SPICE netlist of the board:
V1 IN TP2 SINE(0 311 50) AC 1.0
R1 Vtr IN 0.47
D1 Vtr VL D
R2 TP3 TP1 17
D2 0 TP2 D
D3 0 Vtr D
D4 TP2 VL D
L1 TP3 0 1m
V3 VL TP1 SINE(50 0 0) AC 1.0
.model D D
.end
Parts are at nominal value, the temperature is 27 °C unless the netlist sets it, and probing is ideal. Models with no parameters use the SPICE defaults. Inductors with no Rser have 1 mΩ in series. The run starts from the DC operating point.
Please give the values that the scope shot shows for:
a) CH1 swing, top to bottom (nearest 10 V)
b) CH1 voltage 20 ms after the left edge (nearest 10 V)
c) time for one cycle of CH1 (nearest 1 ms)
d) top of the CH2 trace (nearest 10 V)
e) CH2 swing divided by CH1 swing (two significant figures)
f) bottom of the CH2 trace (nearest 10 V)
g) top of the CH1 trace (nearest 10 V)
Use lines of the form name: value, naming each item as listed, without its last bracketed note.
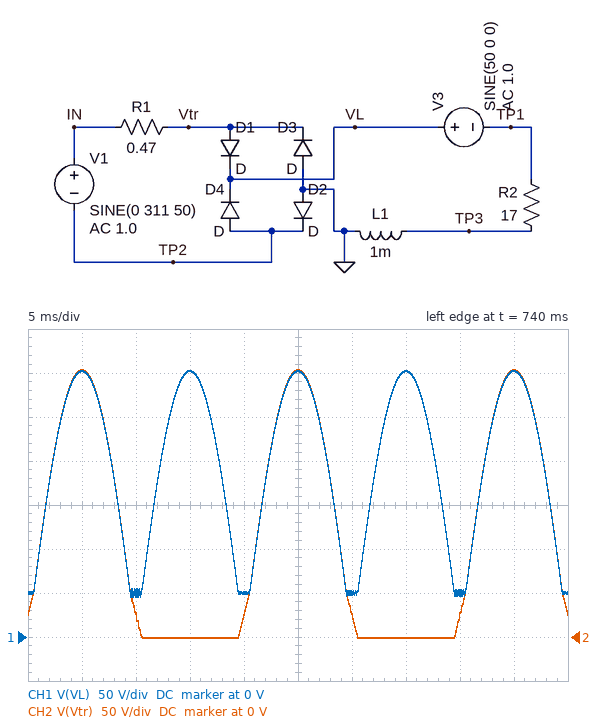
CH1 swing, top to bottom: 260 V
CH1 voltage 20 ms after the left edge: 50 V
time for one cycle of CH1: 10 ms
top of the CH2 trace: 300 V
CH2 swing divided by CH1 swing: 1.2
bottom of the CH2 trace: 0 V
top of the CH1 trace: 300 V
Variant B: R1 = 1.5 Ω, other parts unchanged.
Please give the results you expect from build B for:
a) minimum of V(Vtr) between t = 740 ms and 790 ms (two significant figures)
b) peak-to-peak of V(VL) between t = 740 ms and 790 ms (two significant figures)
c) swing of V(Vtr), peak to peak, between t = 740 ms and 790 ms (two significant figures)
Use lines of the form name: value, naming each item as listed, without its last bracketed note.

minimum of V(Vtr) between t = 740 ms and 790 ms: -900 mV
peak-to-peak of V(VL) between t = 740 ms and 790 ms: 240 V
swing of V(Vtr), peak to peak, between t = 740 ms and 790 ms: 290 V
